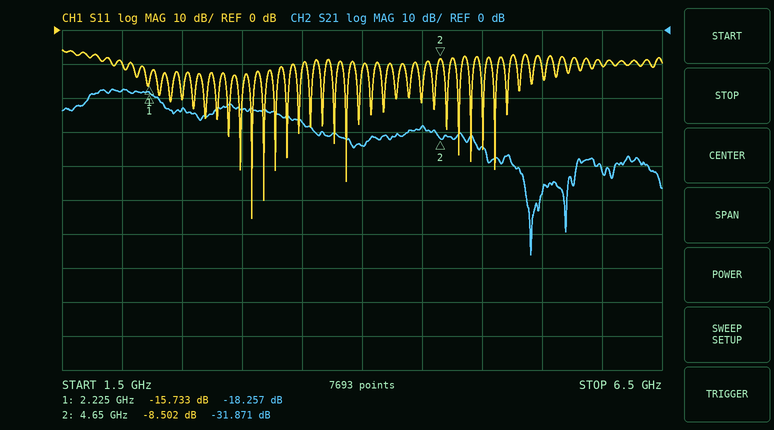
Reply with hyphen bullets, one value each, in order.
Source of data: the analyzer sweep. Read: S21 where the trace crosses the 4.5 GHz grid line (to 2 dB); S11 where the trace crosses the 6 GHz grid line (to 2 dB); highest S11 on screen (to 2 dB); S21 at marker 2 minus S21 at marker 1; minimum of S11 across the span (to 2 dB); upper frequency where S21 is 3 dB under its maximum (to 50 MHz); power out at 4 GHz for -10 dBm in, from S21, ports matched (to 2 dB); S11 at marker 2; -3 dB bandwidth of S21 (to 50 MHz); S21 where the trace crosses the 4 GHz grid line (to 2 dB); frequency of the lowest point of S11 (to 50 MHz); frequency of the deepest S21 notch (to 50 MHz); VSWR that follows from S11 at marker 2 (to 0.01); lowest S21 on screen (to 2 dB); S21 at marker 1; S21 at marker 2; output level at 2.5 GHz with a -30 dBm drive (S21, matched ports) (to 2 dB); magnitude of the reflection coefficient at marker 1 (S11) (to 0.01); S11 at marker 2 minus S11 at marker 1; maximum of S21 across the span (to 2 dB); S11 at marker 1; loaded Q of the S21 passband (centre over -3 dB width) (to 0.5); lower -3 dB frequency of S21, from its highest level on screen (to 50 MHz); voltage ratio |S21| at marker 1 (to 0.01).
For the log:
- -28 dB
- -10 dB
- -6 dB
- -13.614 dB
- -56 dB
- 2.30 GHz
- -44 dBm
- -8.502 dB
- 600 MHz
- -34 dB
- 3.10 GHz
- 5.40 GHz
- 2.20
- -66 dB
- -18.257 dB
- -31.871 dB
- -54 dBm
- 0.16
- 7.231 dB
- -18 dB
- -15.733 dB
- 3.5
- 1.70 GHz
- 0.12
